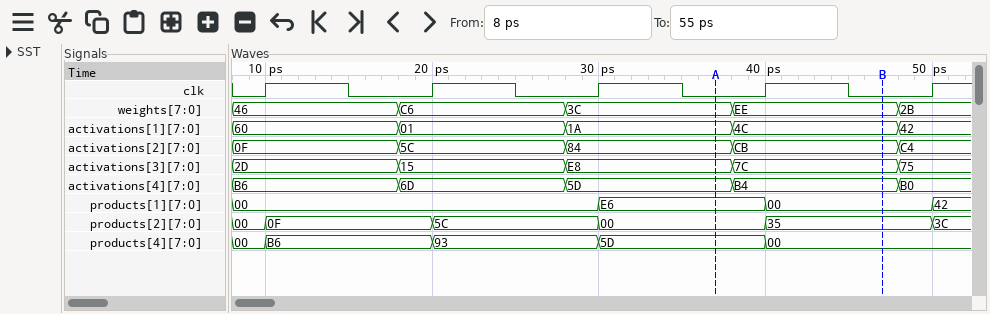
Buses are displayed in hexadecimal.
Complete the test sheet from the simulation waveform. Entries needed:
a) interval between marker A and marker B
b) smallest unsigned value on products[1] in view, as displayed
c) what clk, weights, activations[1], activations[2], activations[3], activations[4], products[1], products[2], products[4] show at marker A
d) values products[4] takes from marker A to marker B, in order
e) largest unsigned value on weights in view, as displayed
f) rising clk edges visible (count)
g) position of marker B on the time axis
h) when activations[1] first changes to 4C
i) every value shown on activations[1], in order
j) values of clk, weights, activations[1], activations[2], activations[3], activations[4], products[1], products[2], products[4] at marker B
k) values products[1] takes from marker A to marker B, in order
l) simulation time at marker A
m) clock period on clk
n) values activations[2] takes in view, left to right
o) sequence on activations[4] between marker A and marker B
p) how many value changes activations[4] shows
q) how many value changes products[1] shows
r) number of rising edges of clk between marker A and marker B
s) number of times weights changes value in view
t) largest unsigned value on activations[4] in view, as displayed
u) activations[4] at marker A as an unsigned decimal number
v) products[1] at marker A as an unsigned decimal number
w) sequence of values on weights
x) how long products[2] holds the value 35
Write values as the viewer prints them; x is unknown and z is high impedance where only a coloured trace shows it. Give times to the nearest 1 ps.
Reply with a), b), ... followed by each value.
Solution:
a) 10 ps
b) 00
c) clk=0, weights=3C, activations[1]=1A, activations[2]=84, activations[3]=E8, activations[4]=5D, products[1]=E6, products[2]=00, products[4]=5D
d) 5D, 00
e) EE
f) 5
g) 47 ps
h) 38 ps
i) 60, 01, 1A, 4C, 42
j) clk=0, weights=EE, activations[1]=4C, activations[2]=CB, activations[3]=7C, activations[4]=B4, products[1]=00, products[2]=35, products[4]=00
k) E6, 00
l) 37 ps
m) 10 ps
n) 0F, 5C, 84, CB, C4
o) 5D, B4
p) 4
q) 3
r) 1
s) 4
t) B6
u) 93
v) 230
w) 46, C6, 3C, EE, 2B
x) 10 ps
